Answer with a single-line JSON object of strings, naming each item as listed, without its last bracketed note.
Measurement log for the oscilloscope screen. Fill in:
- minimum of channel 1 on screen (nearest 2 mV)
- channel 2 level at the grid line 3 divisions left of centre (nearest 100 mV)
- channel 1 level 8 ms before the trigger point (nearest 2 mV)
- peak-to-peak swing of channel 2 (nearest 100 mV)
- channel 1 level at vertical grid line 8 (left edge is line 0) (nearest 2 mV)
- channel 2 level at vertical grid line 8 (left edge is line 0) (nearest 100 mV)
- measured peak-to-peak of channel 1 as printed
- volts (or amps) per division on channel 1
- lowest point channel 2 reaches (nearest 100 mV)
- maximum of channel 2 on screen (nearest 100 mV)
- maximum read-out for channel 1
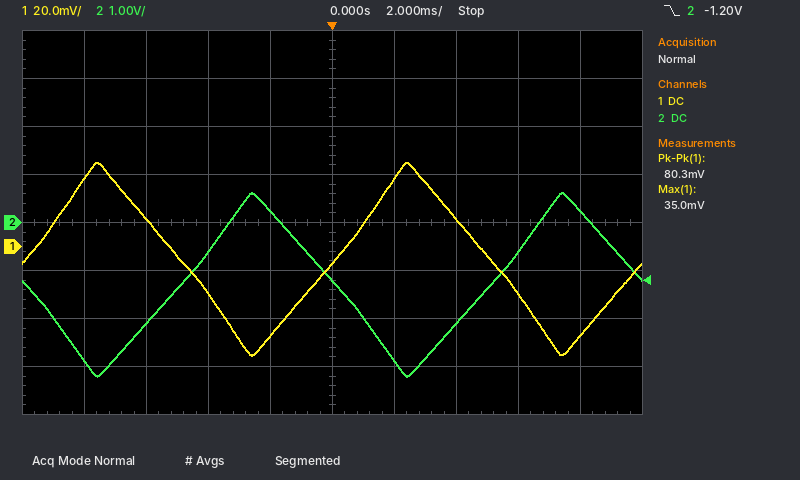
{"minimum of channel 1 on screen": "-46 mV", "channel 2 level at the grid line 3 divisions left of centre": "-2.1 V", "channel 1 level 8 ms before the trigger point": "28 mV", "peak-to-peak swing of channel 2": "3.8 V", "channel 1 level at vertical grid line 8 (left edge is line 0)": "-20 mV", "channel 2 level at vertical grid line 8 (left edge is line 0)": "-600 mV", "measured peak-to-peak of channel 1 as printed": "80.3 mV", "volts (or amps) per division on channel 1": "20 mV", "lowest point channel 2 reaches": "-3.2 V", "maximum of channel 2 on screen": "600 mV", "maximum read-out for channel 1": "35.0 mV"}
